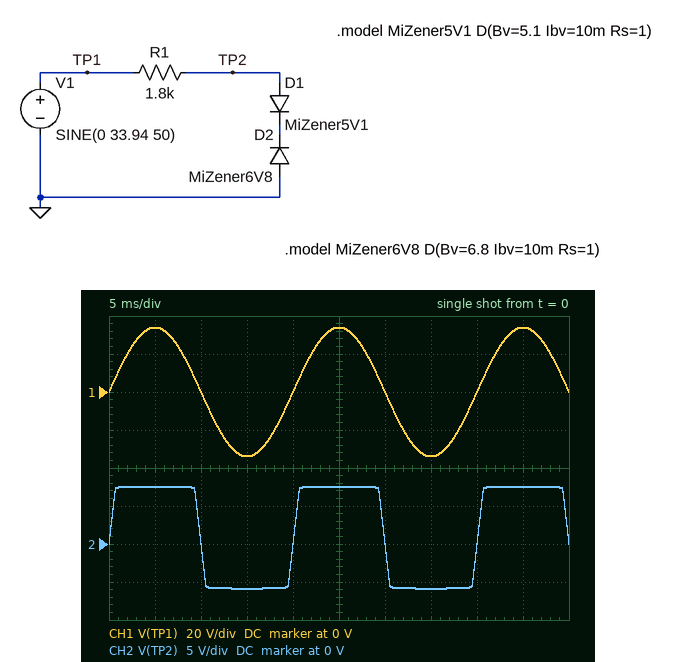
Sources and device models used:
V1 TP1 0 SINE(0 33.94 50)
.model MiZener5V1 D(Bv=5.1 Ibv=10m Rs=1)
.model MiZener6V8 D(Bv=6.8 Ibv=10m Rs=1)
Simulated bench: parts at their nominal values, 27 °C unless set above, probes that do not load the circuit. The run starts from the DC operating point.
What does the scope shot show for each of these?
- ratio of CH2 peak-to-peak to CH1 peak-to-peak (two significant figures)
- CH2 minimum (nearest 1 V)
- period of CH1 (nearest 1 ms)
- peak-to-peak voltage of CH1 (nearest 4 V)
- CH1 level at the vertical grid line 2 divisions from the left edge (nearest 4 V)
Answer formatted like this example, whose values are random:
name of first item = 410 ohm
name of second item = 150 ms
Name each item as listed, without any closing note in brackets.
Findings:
ratio of CH2 peak-to-peak to CH1 peak-to-peak = 0.20
CH2 minimum = -6 V
period of CH1 = 20 ms
peak-to-peak voltage of CH1 = 68 V
CH1 level at the vertical grid line 2 divisions from the left edge = 0 V
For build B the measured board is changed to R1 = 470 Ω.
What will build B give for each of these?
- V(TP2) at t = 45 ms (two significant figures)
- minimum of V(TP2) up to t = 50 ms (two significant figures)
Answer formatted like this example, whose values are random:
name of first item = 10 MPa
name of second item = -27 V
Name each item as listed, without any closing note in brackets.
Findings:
V(TP2) at t = 45 ms = 7.7 V
minimum of V(TP2) up to t = 50 ms = -6.0 V
